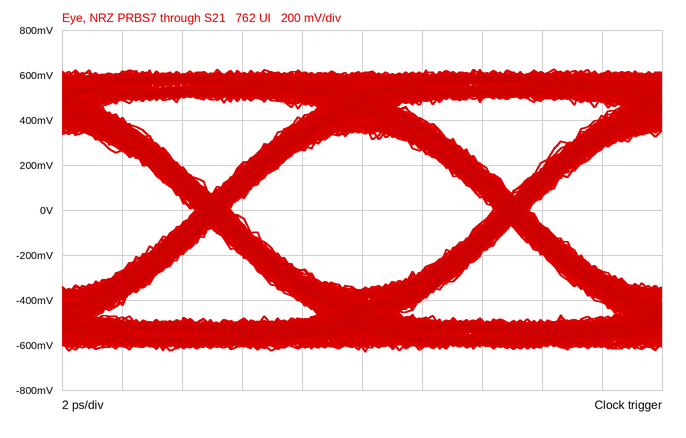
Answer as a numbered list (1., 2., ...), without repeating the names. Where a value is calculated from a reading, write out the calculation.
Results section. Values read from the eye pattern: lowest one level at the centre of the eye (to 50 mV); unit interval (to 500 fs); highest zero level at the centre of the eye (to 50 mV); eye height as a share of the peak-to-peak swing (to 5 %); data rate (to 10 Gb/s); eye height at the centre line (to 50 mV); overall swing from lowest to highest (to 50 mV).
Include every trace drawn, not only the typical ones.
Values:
1. 350 mV
2. 10.0 ps
3. -350 mV
4. 700 mV / 1.25 V ≈ 56.0 %, so 55 % to the nearest 5 %
5. 100 Gb/s
6. 700 mV
7. 1.25 V
